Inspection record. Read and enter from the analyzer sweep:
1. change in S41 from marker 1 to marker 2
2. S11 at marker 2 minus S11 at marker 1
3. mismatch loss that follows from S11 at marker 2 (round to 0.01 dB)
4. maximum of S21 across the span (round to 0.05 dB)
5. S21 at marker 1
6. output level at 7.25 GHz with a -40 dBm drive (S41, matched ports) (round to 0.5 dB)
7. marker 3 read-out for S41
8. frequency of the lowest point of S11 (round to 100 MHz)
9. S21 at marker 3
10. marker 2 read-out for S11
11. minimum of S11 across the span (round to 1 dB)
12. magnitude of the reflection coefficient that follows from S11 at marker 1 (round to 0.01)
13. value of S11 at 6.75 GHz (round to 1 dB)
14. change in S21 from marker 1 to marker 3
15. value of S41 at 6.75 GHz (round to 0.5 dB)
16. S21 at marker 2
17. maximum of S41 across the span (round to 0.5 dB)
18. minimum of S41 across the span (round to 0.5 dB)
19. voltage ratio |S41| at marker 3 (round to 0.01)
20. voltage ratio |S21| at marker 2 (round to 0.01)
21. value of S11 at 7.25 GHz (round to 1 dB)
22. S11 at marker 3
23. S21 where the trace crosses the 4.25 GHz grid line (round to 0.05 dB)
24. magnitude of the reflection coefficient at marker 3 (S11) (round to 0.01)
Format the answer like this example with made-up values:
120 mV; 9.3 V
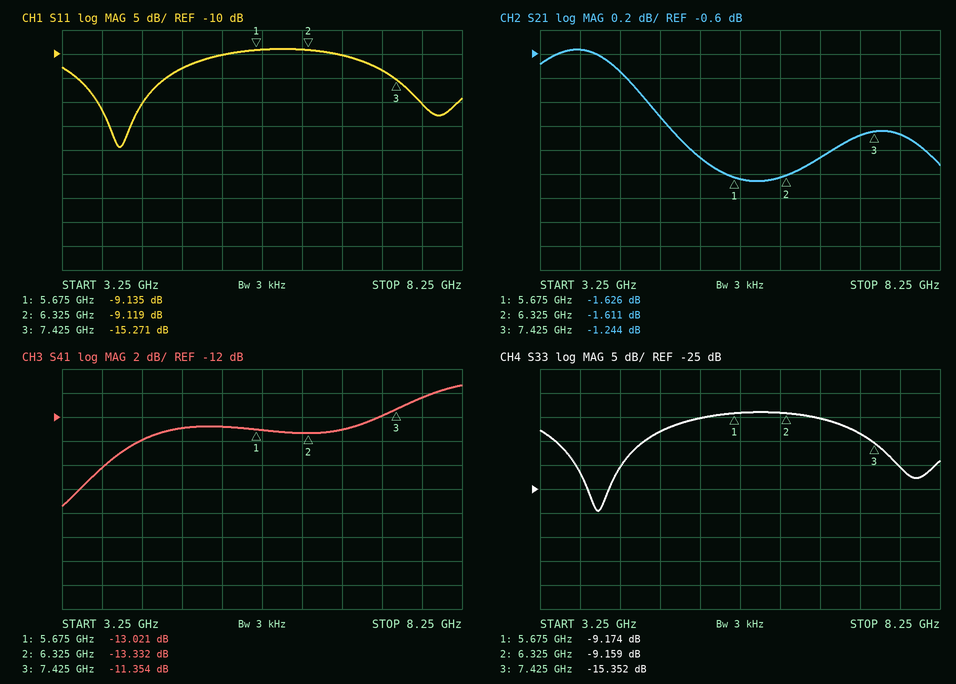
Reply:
-0.311 dB; 0.016 dB; 0.57 dB; -0.55 dB; -1.626 dB; -52.0 dBm; -11.354 dB; 4.0 GHz; -1.244 dB; -9.119 dB; -29 dB; 0.35; -10 dB; 0.382 dB; -13.0 dB; -1.611 dB; -9.5 dB; -19.5 dB; 0.27; 0.83; -13 dB; -15.271 dB; -0.75 dB; 0.17
